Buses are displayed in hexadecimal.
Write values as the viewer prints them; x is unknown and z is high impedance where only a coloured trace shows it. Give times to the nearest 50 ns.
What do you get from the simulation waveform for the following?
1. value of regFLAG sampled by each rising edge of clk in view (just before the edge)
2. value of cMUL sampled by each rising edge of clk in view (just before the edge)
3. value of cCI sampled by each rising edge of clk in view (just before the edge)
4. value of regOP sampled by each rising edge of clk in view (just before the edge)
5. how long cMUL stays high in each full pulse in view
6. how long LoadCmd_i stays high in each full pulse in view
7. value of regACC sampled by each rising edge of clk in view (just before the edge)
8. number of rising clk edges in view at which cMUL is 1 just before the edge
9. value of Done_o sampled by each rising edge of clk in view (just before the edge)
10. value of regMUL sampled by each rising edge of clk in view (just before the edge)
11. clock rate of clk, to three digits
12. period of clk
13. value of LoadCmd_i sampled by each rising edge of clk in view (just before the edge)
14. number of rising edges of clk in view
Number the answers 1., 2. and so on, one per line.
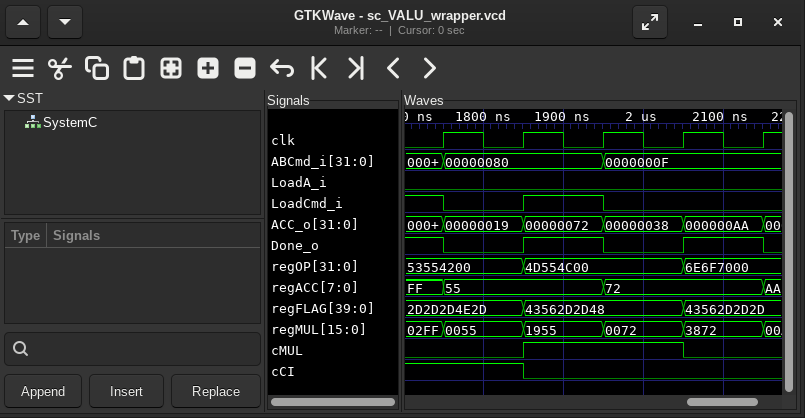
1. 2D2D2D4E2D, 2D2D2D4E2D, 43562D2D48, 43562D2D48, 43562D2D2D
2. 0 0 1 1 0
3. 1 1 0 0 0
4. 53554200, 53554200, 4D554C00, 4D554C00, 6E6F7000
5. 200 ns
6. 100 ns
7. FF, 55, 55, 72, 72
8. 2
9. 1 0 1 0 1
10. 02FF, 0055, 1955, 0072, 3872
11. 10.0 MHz
12. 100 ns
13. 1 0 1 0 0
14. 5
